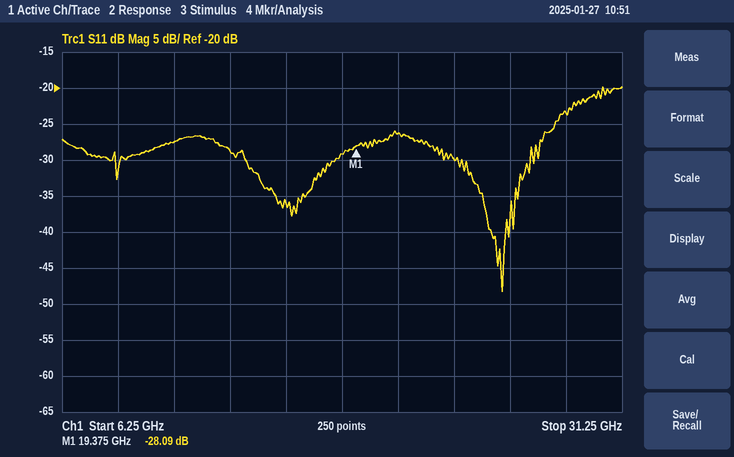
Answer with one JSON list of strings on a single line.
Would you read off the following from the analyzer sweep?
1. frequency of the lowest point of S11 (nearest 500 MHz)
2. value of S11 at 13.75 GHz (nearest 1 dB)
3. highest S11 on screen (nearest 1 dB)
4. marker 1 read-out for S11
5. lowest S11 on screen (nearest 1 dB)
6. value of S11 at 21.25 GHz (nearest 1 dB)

["26.0 GHz", "-29 dB", "-20 dB", "-28.09 dB", "-48 dB", "-26 dB"]
